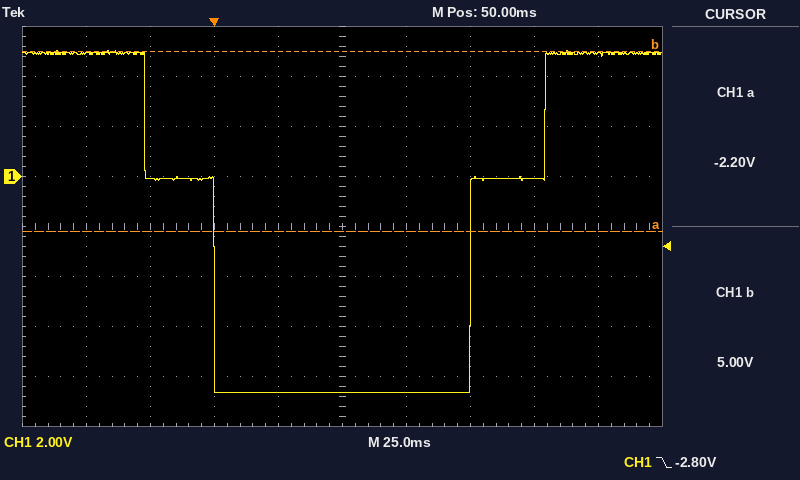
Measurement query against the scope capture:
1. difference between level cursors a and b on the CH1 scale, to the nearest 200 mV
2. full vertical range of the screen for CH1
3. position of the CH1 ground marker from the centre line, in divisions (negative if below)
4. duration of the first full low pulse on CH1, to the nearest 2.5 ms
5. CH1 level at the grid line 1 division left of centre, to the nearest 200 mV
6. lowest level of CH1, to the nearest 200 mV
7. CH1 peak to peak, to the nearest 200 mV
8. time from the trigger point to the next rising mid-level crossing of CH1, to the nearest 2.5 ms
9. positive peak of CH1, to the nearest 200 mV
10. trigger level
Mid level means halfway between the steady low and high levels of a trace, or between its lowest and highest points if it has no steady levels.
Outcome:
7.2 V
16 V
+1.0 div
100.0 ms
-8.6 V
-8.6 V
13.6 V
100.0 ms
5.0 V
-2.80 V
